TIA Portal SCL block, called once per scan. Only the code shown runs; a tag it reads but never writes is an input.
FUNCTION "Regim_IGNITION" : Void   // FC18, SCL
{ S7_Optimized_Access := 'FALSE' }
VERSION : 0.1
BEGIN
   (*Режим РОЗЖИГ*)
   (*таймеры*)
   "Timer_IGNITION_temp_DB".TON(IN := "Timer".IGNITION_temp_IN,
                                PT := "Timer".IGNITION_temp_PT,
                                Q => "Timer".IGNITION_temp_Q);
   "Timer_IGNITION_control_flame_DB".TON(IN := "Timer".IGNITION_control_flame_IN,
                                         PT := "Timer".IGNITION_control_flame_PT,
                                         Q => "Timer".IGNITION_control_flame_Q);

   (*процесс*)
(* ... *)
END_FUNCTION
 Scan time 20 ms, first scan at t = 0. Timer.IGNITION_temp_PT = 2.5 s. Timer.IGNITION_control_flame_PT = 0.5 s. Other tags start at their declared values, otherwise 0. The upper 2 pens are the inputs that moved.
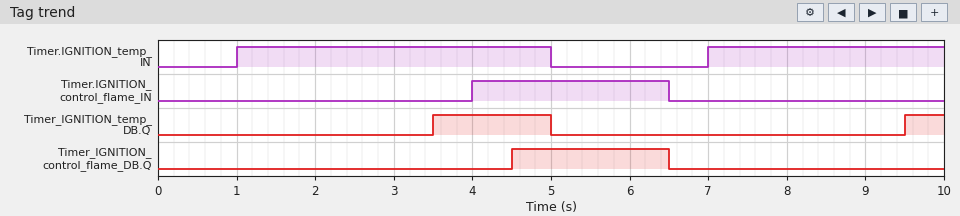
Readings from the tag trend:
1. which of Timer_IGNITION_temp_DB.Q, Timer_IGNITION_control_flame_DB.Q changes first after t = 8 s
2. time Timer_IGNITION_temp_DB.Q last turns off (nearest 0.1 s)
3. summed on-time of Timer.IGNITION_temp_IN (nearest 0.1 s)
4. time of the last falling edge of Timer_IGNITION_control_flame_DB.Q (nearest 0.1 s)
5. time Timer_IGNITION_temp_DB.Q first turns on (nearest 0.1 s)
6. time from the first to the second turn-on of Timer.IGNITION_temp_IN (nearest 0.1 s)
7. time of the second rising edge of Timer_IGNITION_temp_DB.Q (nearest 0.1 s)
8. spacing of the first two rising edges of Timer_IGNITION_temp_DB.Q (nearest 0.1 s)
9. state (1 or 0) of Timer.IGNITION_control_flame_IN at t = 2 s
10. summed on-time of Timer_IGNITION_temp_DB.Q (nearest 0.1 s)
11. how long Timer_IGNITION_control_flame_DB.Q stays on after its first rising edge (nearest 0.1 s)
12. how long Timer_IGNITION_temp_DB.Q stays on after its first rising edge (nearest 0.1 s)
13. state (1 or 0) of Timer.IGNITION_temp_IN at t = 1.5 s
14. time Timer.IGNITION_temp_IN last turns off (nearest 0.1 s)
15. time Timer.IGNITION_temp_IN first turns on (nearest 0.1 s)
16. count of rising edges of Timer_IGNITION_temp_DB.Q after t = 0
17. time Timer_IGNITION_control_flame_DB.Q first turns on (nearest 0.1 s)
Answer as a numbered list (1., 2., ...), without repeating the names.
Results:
1. Timer_IGNITION_temp_DB.Q
2. 5.0 s
3. 7.0 s
4. 6.5 s
5. 3.5 s
6. 6.0 s
7. 9.5 s
8. 6.0 s
9. 0
10. 2.0 s
11. 2.0 s
12. 1.5 s
13. 1
14. 5.0 s
15. 1.0 s
16. 2
17. 4.5 s
